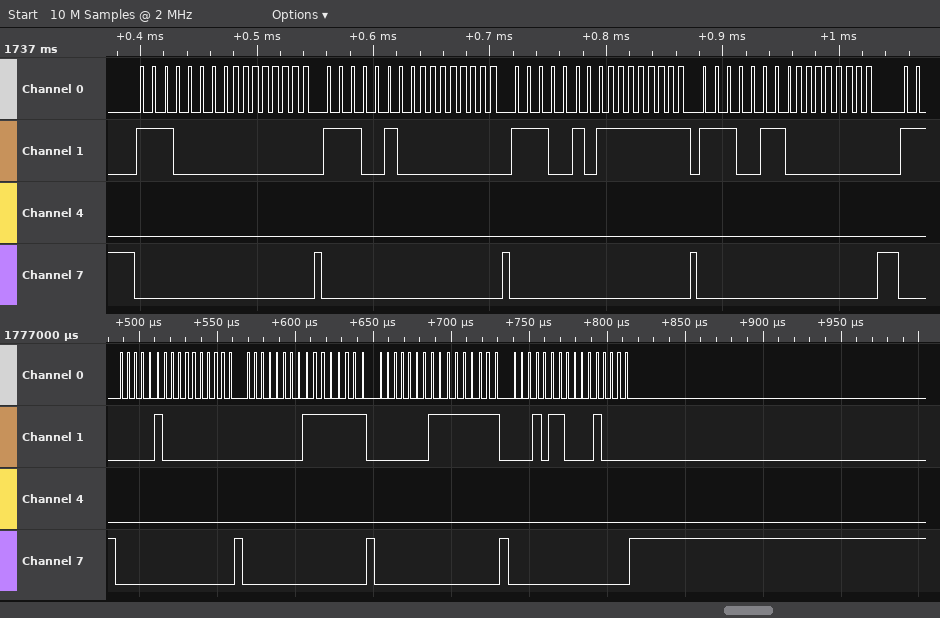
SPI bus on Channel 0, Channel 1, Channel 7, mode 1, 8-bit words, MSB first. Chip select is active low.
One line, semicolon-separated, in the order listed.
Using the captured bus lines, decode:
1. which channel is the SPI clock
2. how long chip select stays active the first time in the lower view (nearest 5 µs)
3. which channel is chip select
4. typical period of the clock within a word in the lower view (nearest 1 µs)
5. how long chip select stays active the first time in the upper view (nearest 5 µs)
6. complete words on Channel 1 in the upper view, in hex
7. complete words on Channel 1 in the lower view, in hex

Channel 0; 75 µs; Channel 7; 5 µs; 155 µs; E0, 00, E4, 00, E5, FF, E6, 00; 04, 00, 00, FF, 01, FF, 16, 10
